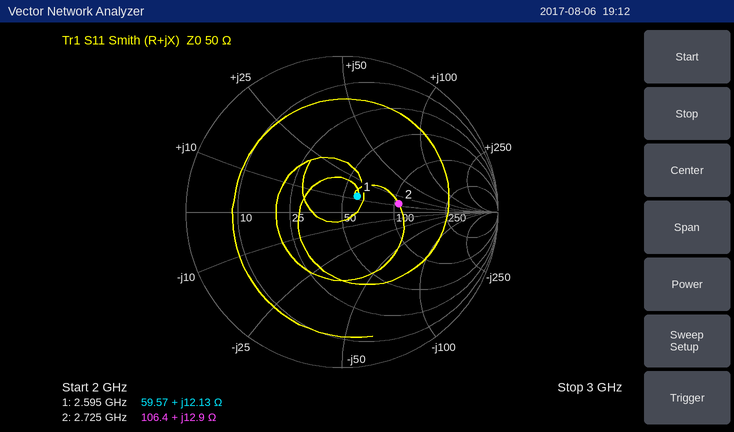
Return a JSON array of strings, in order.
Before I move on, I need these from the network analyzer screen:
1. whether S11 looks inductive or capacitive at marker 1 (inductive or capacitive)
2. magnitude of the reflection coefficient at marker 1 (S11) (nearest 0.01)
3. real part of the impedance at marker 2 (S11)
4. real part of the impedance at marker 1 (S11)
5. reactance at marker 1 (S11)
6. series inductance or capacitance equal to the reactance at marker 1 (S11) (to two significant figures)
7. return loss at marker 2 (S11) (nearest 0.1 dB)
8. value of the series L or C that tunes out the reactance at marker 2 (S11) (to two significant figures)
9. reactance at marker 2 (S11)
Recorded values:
["inductive", "0.14", "106.4 Ω", "59.57 Ω", "+12.13 Ω", "740 pH", "8.7 dB", "4.5 pF", "+12.9 Ω"]
